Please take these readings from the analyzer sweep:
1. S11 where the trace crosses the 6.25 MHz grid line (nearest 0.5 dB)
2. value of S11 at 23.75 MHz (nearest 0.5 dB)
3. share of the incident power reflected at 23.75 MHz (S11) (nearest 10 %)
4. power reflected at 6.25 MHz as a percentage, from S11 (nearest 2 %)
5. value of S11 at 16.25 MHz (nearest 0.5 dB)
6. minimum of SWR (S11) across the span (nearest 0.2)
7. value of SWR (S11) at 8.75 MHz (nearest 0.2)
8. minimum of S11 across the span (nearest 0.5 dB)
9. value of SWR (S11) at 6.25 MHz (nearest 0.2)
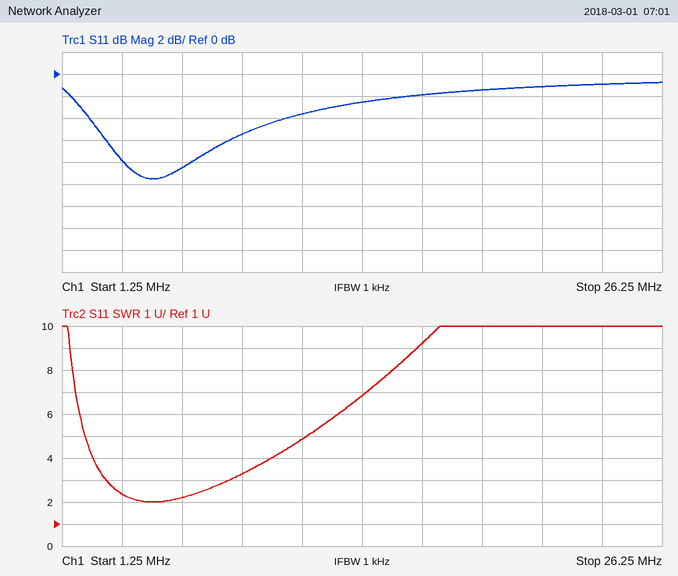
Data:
-8.5 dB
-1.0 dB
80 %
14 %
-2.0 dB
2.0
3.2
-9.5 dB
2.2
